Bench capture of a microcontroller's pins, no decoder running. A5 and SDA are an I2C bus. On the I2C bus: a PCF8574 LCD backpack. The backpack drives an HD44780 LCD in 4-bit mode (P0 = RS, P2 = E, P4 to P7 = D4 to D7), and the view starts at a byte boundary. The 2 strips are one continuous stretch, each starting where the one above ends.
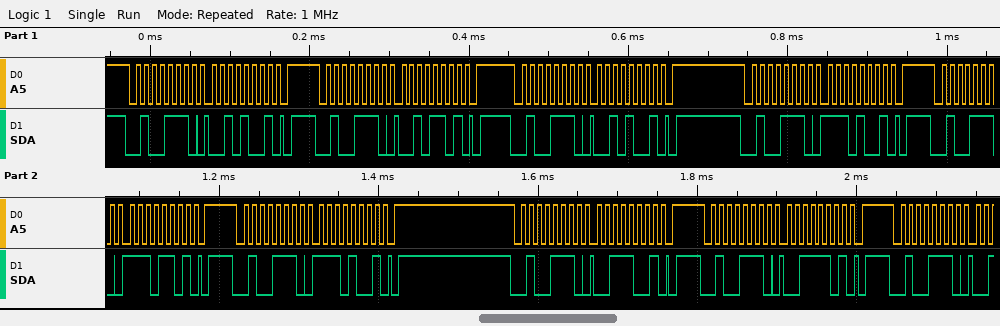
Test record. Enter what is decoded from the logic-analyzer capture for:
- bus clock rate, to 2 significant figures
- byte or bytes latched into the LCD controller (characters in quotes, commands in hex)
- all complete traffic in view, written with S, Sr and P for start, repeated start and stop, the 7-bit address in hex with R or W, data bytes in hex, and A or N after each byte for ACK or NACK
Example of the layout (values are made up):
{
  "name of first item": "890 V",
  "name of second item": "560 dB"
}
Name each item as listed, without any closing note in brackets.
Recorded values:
{
  "bus clock rate, to 2 significant figures": "100 kHz",
  "byte or bytes latched into the LCD controller": "'.'",
  "all complete traffic in view, written with S, Sr and P for start, repeated start and stop, the 7-bit address in hex with R or W, data bytes in hex, and A or N after each byte for ACK or NACK": "S 27W A 29 A P S 27W A 2D A P S 27W A 29 A P S 27W A E9 A P S 27W A ED A P S 27W A E9 A P S 27W A 39 A P S 27W A 3D A P S 27W A"
}
